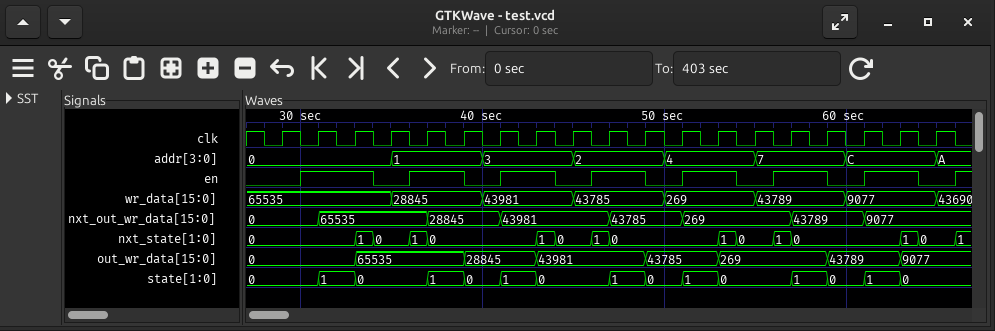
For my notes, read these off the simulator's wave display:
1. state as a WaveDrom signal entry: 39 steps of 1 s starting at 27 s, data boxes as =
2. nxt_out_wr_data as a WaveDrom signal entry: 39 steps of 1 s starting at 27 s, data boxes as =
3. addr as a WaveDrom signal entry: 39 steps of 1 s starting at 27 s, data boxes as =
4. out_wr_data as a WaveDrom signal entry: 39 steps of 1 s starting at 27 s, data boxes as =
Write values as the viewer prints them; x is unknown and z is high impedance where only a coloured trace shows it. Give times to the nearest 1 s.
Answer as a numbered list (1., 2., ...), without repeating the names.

1. {name: 'state', wave: '=...=.=...=.=.=.=...=.=.=.=...=.=.=.=..', data: '0 1 0 1 0 1 0 1 0 1 0 1 0 1 0'}
2. {name: 'nxt_out_wr_data', wave: '=...=.....=...=.....=...=.....=...=....', data: '0 65535 28845 43981 43785 269 43789 9077'}
3. {name: 'addr', wave: '=.......=....=....=....=....=....=....=', data: '0 1 3 2 4 7 C A'}
4. {name: 'out_wr_data', wave: '=.....=.....=...=.....=...=.....=...=..', data: '0 65535 28845 43981 43785 269 43789 9077'}
